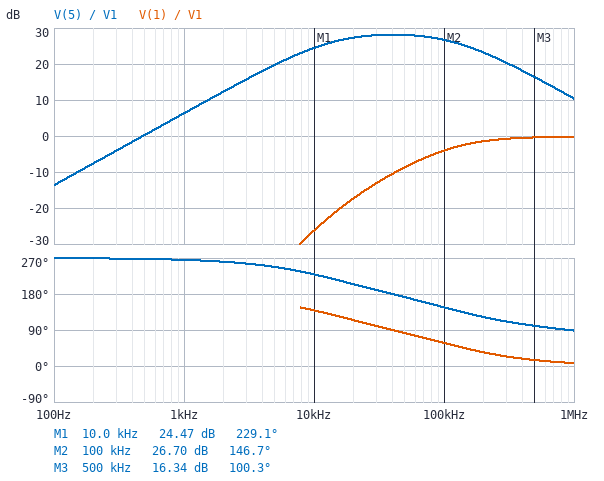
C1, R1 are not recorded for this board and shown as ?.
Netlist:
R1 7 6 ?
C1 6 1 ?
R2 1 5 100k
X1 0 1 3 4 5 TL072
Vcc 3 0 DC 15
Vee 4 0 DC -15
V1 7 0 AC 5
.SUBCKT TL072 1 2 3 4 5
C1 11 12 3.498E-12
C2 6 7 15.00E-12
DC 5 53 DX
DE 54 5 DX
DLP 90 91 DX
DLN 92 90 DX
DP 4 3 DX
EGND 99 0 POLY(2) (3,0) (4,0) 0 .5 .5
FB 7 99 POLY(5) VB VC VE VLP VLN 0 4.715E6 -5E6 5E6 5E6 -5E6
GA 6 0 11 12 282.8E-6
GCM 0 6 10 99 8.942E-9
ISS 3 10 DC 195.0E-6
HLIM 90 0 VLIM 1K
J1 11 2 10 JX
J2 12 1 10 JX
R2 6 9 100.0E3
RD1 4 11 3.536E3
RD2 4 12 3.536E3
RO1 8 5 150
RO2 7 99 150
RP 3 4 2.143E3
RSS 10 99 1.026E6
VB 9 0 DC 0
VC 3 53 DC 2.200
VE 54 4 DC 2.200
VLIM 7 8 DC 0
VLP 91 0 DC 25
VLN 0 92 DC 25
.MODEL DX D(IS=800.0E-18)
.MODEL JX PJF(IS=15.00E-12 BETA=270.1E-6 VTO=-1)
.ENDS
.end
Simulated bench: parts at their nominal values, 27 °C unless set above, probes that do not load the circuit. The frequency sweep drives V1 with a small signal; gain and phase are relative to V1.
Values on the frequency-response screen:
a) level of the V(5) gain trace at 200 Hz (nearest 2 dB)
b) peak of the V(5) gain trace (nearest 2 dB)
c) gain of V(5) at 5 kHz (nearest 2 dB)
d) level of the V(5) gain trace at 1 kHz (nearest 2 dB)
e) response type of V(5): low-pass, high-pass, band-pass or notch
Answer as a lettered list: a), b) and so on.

a) -8 dB
b) 28 dB
c) 20 dB
d) 6 dB
e) band-pass
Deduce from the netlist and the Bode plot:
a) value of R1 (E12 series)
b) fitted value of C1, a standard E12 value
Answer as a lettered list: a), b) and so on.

a) 3.9 kΩ
b) 3.3 nF
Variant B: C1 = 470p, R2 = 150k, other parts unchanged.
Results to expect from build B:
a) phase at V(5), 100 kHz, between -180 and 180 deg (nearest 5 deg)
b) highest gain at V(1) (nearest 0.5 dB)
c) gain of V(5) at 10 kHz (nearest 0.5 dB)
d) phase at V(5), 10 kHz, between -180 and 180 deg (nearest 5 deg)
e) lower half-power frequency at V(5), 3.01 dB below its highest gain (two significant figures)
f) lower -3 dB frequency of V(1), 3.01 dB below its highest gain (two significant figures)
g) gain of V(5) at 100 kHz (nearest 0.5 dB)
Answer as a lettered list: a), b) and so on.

a) 165 deg
b) 1.0 dB
c) 13.0 dB
d) -95 deg
e) 54 kHz
f) 75 kHz
g) 31.5 dB
